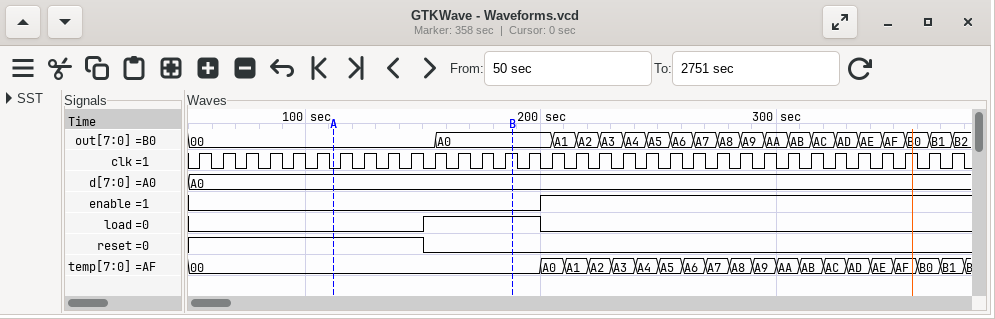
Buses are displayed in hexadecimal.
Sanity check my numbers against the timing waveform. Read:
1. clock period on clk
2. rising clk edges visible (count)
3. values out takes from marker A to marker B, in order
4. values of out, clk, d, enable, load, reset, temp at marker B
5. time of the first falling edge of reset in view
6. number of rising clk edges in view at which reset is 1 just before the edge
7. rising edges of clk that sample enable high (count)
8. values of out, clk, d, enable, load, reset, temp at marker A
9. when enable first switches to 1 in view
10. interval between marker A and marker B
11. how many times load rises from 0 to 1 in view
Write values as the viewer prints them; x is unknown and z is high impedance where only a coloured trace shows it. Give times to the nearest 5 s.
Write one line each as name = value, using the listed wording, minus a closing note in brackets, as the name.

clock period on clk = 10 s
rising clk edges visible = 33
values out takes from marker A to marker B, in order = 00, A0
values of out, clk, d, enable, load, reset, temp at marker B = out=A0, clk=1, d=A0, enable=0, load=1, reset=0, temp=00
time of the first falling edge of reset in view = 150 s
number of rising clk edges in view at which reset is 1 just before the edge = 10
rising edges of clk that sample enable high = 18
values of out, clk, d, enable, load, reset, temp at marker A = out=00, clk=0, d=A0, enable=0, load=0, reset=1, temp=00
when enable first switches to 1 in view = 200 s
interval between marker A and marker B = 75 s
how many times load rises from 0 to 1 in view = 1
